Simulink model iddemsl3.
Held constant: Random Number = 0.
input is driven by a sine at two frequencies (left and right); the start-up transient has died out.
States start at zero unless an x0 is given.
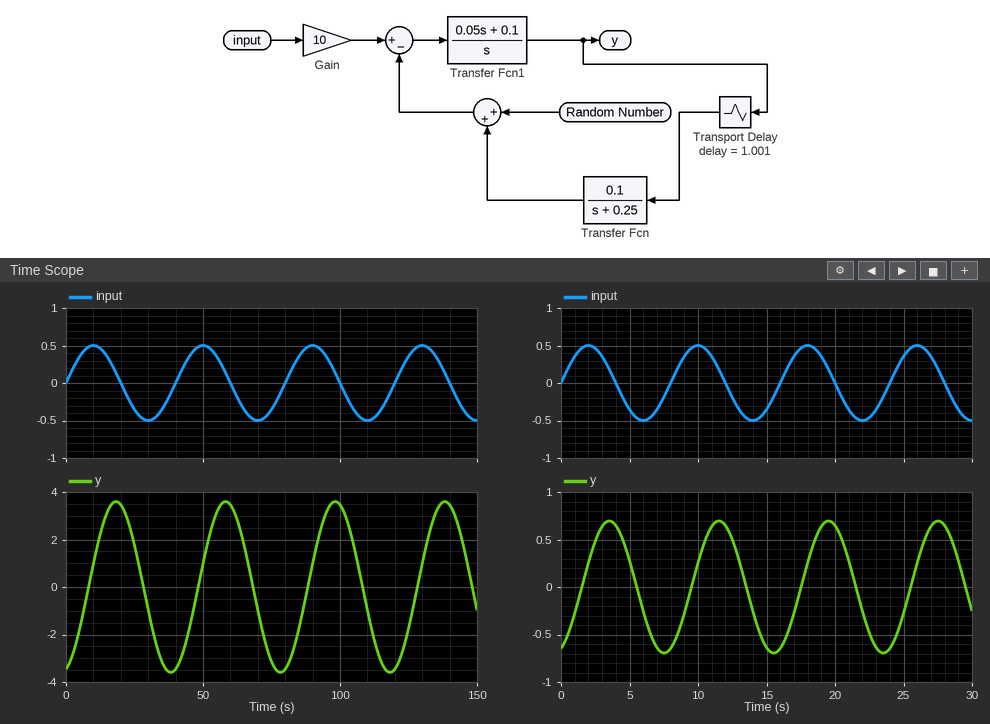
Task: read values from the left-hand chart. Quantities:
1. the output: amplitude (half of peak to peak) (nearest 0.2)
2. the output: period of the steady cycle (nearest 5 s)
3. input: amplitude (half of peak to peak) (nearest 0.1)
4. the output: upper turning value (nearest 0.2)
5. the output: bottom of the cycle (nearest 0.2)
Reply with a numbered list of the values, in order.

1. 3.6
2. 40 s
3. 0.5
4. 3.6
5. -3.6
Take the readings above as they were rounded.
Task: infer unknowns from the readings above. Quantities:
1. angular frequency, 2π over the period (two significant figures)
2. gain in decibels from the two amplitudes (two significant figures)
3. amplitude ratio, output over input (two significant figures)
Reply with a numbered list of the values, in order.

1. 0.16 rad/s
2. 17 dB
3. 7.2
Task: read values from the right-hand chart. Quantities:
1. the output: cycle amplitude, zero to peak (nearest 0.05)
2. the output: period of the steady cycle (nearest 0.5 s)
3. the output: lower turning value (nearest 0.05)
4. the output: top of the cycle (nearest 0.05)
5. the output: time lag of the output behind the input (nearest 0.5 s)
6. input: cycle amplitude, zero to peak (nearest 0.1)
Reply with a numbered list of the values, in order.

1. 0.70
2. 8.0 s
3. -0.70
4. 0.70
5. 1.5 s
6. 0.5
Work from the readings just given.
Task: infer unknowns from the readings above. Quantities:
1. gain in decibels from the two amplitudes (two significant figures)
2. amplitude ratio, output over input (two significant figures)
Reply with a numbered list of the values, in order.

1. 2.9 dB
2. 1.4
